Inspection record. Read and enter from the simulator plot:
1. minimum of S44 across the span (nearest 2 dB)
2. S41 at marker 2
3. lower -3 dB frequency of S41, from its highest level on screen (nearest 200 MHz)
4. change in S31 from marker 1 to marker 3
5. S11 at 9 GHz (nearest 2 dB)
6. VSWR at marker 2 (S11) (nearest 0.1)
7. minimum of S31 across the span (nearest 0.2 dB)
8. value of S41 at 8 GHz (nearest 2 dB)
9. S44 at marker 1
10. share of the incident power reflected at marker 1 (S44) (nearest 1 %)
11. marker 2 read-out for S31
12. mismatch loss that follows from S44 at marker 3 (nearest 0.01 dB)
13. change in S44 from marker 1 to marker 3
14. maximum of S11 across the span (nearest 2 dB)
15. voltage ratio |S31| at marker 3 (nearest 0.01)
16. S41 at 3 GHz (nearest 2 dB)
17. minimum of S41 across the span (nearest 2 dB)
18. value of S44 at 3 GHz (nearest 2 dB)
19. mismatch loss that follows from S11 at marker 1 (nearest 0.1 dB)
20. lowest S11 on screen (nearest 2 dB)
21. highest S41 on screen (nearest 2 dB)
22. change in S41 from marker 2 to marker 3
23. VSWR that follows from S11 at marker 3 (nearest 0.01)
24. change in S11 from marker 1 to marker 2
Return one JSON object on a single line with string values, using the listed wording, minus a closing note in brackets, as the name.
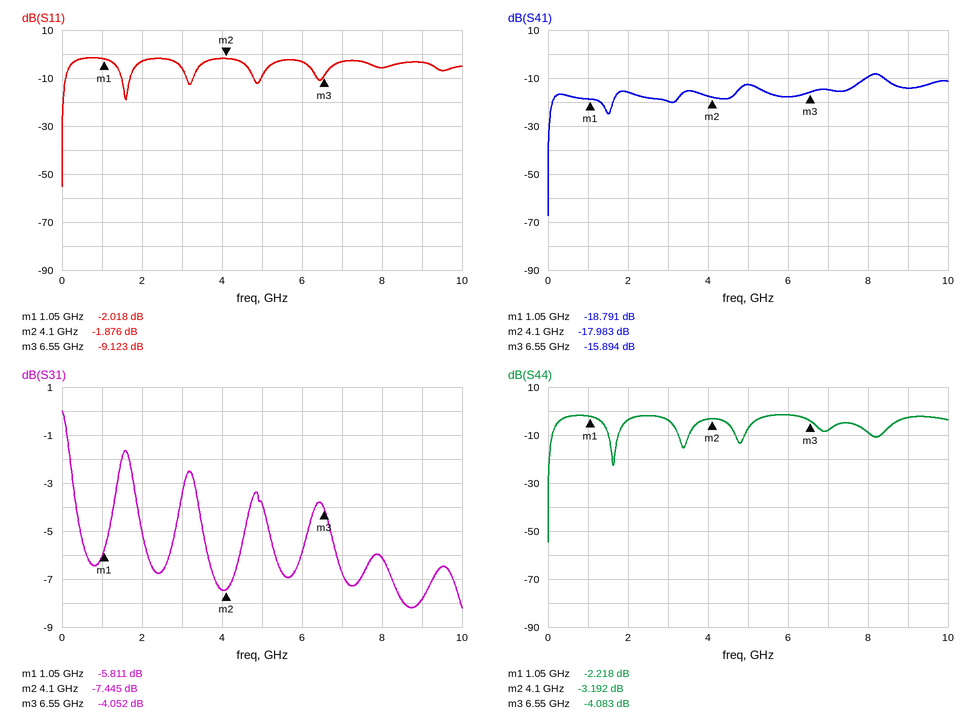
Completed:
{"minimum of S44 across the span": "-54 dB", "S41 at marker 2": "-17.983 dB", "lower -3 dB frequency of S41, from its highest level on screen": "7.8 GHz", "change in S31 from marker 1 to marker 3": "1.759 dB", "S11 at 9 GHz": "-4 dB", "VSWR at marker 2 (S11)": "9.3", "minimum of S31 across the span": "-8.2 dB", "value of S41 at 8 GHz": "-10 dB", "S44 at marker 1": "-2.218 dB", "share of the incident power reflected at marker 1 (S44)": "60 %", "marker 2 read-out for S31": "-7.445 dB", "mismatch loss that follows from S44 at marker 3": "2.15 dB", "change in S44 from marker 1 to marker 3": "-1.865 dB", "maximum of S11 across the span": "-2 dB", "voltage ratio |S31| at marker 3": "0.63", "S41 at 3 GHz": "-20 dB", "minimum of S41 across the span": "-68 dB", "value of S44 at 3 GHz": "-4 dB", "mismatch loss that follows from S11 at marker 1": "4.3 dB", "lowest S11 on screen": "-56 dB", "highest S41 on screen": "-8 dB", "change in S41 from marker 2 to marker 3": "2.089 dB", "VSWR that follows from S11 at marker 3": "2.08", "change in S11 from marker 1 to marker 2": "0.142 dB"}
